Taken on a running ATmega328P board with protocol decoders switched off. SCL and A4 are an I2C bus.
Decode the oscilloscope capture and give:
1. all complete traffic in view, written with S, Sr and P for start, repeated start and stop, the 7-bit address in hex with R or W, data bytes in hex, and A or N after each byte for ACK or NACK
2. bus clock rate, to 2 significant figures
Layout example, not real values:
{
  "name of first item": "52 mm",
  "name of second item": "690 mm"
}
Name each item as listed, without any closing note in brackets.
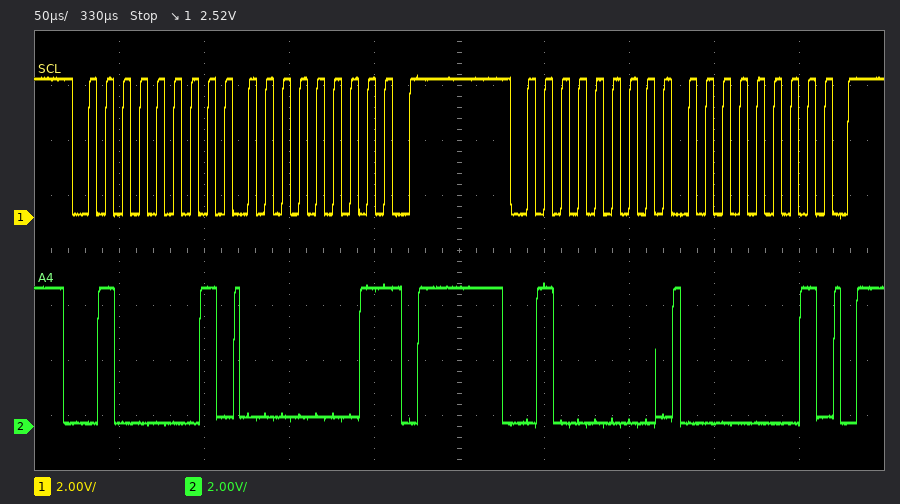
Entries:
{
  "all complete traffic in view, written with S, Sr and P for start, repeated start and stop, the 7-bit address in hex with R or W, data bytes in hex, and A or N after each byte for ACK or NACK": "S 20R A 01 N P S 20W A 01 A P",
  "bus clock rate, to 2 significant figures": "100 kHz"
}
